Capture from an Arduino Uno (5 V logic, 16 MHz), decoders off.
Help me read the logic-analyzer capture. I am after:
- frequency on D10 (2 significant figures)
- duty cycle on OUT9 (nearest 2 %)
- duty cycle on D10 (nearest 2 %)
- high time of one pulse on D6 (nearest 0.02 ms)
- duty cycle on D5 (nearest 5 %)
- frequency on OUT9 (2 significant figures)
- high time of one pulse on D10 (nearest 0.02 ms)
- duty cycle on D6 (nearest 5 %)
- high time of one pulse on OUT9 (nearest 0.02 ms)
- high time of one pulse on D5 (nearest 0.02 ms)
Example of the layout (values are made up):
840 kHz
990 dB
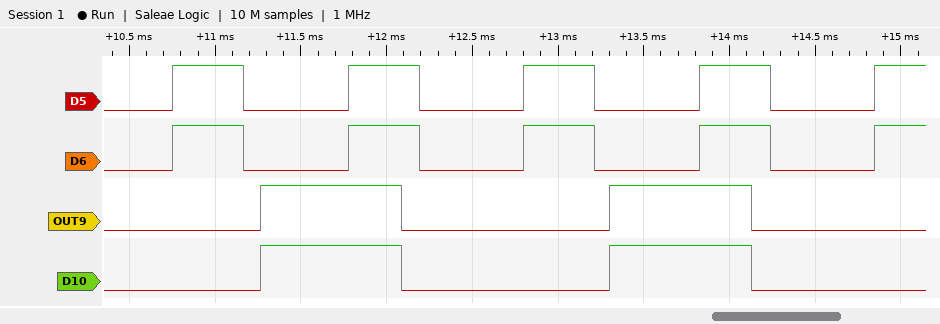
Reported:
490 Hz
40 %
40 %
0.42 ms
40 %
490 Hz
0.82 ms
40 %
0.82 ms
0.42 ms
